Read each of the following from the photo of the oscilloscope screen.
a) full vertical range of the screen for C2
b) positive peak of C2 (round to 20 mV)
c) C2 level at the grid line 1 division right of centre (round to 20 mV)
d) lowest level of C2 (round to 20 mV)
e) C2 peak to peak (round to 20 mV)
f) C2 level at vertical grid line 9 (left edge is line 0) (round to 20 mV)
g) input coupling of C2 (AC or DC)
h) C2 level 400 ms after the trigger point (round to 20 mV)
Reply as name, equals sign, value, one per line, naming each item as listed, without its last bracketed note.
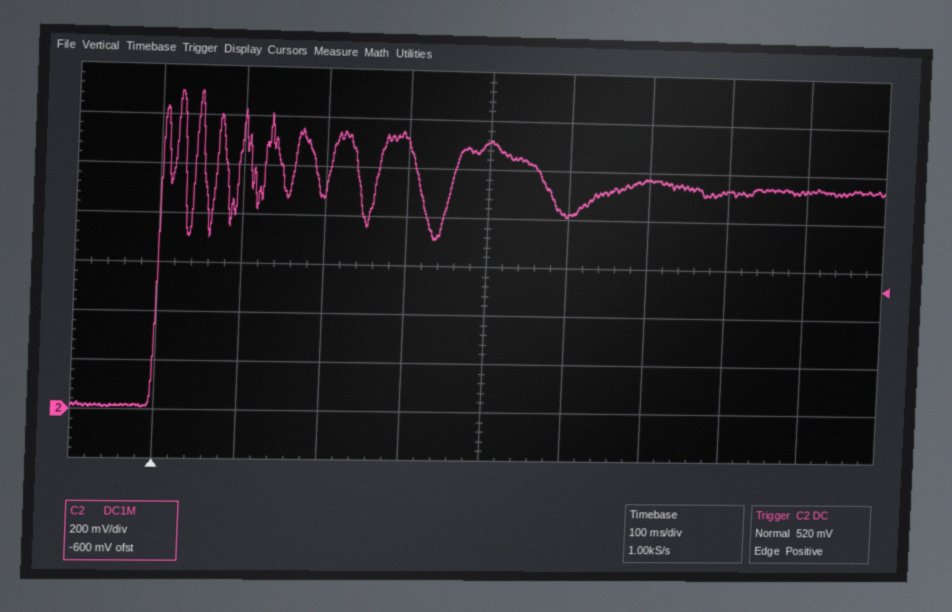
full vertical range of the screen for C2 = 1.6 V
positive peak of C2 = 1.30 V
C2 level at the grid line 1 division right of centre = 820 mV
lowest level of C2 = 20 mV
C2 peak to peak = 1.28 V
C2 level at vertical grid line 9 (left edge is line 0) = 940 mV
input coupling of C2 = DC
C2 level 400 ms after the trigger point = 1.12 V
